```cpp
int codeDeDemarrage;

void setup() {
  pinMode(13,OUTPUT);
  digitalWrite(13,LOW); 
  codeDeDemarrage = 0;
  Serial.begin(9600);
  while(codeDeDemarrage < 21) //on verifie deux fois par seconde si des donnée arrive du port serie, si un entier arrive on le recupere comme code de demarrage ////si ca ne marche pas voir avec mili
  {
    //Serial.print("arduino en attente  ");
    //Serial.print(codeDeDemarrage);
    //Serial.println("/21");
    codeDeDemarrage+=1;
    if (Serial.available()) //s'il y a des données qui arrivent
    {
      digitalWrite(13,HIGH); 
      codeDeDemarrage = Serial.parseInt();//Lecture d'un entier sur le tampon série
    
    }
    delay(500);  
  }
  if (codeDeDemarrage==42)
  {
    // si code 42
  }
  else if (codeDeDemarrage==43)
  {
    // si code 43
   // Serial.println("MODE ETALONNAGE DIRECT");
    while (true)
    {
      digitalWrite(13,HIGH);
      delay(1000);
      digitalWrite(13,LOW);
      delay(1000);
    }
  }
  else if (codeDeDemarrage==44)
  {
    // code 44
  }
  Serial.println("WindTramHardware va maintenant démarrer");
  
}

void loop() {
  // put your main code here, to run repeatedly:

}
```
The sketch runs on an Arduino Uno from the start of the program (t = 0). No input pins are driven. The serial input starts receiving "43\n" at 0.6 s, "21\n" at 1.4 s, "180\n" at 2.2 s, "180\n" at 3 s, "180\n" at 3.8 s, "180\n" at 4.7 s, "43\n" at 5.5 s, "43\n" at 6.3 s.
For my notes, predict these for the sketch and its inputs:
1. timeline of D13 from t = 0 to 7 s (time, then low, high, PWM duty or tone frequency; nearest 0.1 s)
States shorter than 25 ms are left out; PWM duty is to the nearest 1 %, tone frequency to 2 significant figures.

0 s low; 1 s high; 2.5 s low; 3.5 s high; 4.5 s low; 5.5 s high; 6.5 s low
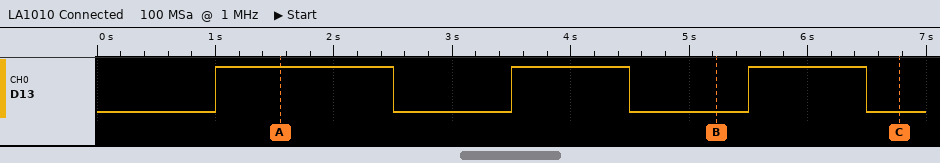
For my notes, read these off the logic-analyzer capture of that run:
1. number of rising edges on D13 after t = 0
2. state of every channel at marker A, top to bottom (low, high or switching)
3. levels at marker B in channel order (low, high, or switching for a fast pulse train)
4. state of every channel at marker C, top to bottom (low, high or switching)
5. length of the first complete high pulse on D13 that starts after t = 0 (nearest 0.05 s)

3
D13 high
D13 low
D13 low
1.50 s
